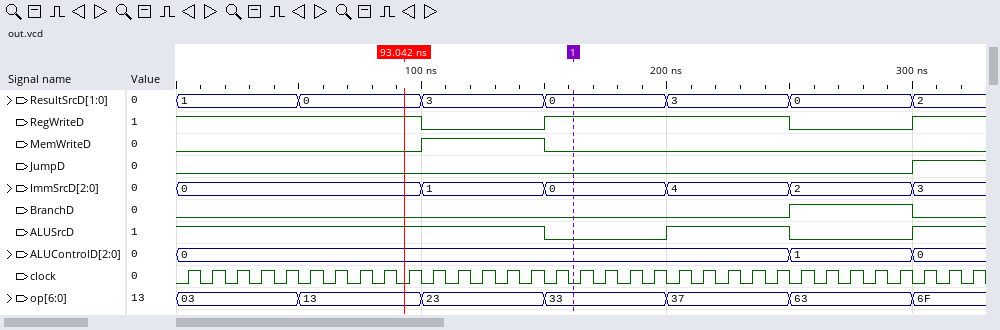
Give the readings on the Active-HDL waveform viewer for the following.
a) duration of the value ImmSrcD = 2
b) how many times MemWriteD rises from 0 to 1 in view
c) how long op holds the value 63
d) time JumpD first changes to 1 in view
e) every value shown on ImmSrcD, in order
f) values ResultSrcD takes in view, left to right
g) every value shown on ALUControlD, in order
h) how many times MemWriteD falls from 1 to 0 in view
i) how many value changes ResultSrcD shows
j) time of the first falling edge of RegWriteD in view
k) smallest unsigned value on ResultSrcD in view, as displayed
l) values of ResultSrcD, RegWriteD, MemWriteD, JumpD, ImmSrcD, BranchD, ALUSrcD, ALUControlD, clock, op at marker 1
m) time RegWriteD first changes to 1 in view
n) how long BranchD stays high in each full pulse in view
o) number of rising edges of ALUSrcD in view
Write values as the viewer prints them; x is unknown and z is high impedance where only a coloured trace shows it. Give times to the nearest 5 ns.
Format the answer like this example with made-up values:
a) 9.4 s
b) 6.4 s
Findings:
a) 50 ns
b) 1
c) 50 ns
d) 300 ns
e) 0, 1, 0, 4, 2, 3
f) 1, 0, 3, 0, 3, 0, 2
g) 0, 1, 0
h) 1
i) 6
j) 100 ns
k) 0
l) ResultSrcD=0, RegWriteD=1, MemWriteD=0, JumpD=0, ImmSrcD=0, BranchD=0, ALUSrcD=0, ALUControlD=0, clock=0, op=33
m) 150 ns
n) 50 ns
o) 2
